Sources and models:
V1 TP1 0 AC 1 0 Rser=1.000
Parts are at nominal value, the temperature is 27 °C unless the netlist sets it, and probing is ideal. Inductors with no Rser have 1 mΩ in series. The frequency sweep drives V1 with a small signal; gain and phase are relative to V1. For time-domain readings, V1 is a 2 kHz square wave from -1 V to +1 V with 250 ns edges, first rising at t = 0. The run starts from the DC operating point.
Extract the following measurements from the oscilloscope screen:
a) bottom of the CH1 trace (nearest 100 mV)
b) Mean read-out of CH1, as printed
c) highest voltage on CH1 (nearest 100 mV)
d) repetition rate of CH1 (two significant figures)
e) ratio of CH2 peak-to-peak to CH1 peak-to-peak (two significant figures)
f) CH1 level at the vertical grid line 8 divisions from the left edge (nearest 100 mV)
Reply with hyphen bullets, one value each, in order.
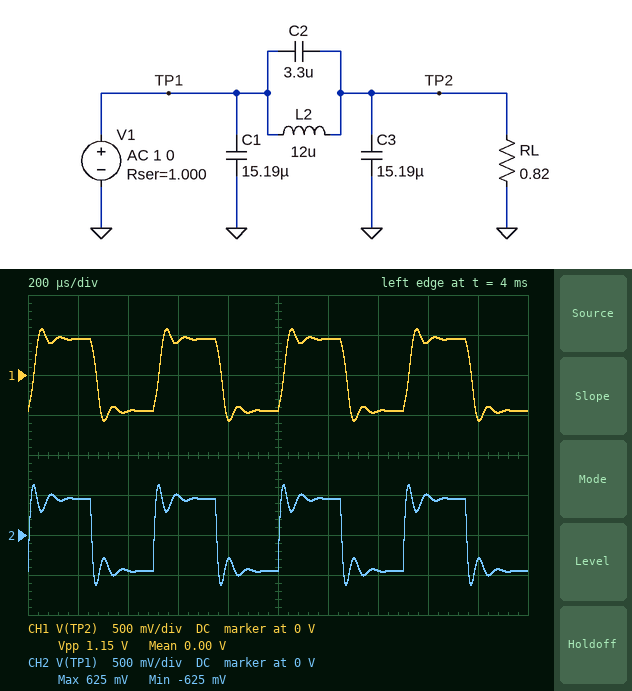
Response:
- -600 mV
- 0.00 V
- 600 mV
- 2.0 kHz
- 1.1
- 400 mV
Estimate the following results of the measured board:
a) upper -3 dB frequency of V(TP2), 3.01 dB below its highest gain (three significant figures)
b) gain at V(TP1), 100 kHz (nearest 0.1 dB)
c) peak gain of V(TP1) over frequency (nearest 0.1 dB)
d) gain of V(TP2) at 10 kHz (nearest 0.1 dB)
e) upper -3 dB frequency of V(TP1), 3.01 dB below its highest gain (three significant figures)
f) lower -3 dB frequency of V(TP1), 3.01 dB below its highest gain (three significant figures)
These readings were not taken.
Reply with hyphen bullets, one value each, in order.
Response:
- 14.3 kHz
- -21.0 dB
- -2.8 dB
- -6.9 dB
- 20.1 kHz
- 10.3 kHz
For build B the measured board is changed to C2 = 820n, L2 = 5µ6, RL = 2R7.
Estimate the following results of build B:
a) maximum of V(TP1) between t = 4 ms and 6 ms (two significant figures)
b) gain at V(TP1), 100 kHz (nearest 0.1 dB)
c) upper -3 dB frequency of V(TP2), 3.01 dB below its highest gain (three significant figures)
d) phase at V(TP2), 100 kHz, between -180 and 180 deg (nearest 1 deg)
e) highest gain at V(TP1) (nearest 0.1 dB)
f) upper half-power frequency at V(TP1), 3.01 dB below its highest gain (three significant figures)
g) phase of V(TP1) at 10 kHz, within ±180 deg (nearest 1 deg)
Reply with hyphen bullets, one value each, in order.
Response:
- 770 mV
- -19.8 dB
- 24.8 kHz
- -82 deg
- -2.4 dB
- 28.6 kHz
- -51 deg
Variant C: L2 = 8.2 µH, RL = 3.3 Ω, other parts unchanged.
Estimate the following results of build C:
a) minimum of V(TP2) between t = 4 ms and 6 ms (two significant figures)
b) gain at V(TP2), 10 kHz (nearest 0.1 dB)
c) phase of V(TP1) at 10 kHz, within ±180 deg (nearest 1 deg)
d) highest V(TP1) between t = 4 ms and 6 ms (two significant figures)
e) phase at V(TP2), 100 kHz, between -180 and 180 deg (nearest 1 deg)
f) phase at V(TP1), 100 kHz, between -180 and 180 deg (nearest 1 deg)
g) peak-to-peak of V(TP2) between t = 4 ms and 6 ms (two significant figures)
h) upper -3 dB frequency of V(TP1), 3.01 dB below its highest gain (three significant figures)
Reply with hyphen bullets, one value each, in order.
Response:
- -850 mV
- -4.4 dB
- -48 deg
- 840 mV
- -83 deg
- -85 deg
- 1.7 V
- 21.3 kHz
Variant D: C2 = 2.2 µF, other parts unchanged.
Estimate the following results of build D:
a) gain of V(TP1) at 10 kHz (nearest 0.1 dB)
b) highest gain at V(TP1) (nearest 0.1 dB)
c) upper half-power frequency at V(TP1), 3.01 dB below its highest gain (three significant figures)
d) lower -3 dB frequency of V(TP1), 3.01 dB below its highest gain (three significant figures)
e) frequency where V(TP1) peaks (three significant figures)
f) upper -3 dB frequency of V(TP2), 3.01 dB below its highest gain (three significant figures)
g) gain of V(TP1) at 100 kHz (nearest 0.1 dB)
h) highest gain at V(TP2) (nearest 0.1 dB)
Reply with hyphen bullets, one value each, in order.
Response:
- -6.5 dB
- -2.9 dB
- 21.5 kHz
- 10.7 kHz
- 15.1 kHz
- 15.3 kHz
- -20.6 dB
- -6.9 dB
